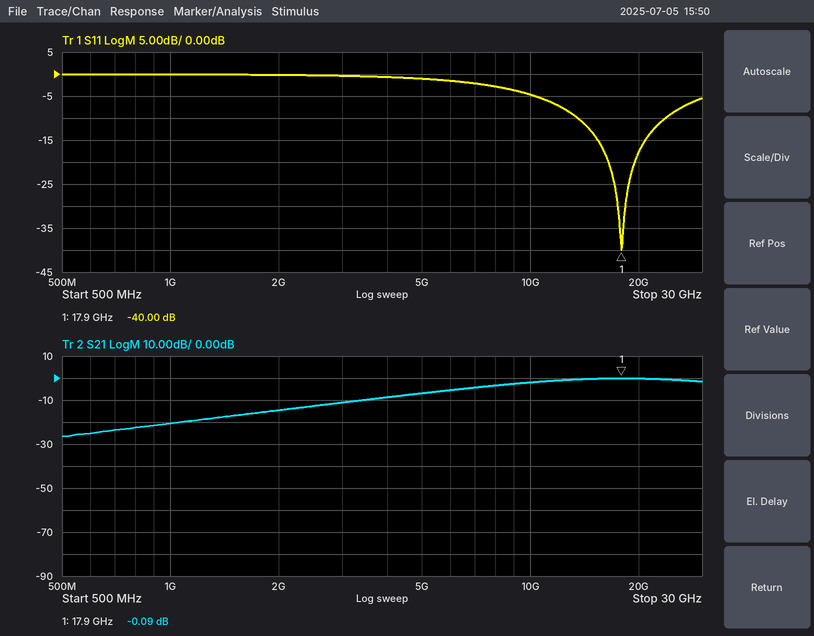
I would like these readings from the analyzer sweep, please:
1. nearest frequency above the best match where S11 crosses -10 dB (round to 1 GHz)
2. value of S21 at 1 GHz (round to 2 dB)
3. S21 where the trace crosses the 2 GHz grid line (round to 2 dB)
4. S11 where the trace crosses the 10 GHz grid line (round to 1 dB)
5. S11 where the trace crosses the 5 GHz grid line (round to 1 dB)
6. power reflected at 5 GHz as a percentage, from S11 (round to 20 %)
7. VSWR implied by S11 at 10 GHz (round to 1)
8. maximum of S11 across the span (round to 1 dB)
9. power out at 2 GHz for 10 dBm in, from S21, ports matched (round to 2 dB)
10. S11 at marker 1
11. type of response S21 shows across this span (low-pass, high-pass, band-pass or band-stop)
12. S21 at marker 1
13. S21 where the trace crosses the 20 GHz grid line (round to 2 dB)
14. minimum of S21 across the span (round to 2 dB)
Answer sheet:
24 GHz
-20 dB
-14 dB
-5 dB
-1 dB
80 %
4
0 dB
-4 dBm
-40.00 dB
high-pass
-0.09 dB
0 dB
-26 dB
